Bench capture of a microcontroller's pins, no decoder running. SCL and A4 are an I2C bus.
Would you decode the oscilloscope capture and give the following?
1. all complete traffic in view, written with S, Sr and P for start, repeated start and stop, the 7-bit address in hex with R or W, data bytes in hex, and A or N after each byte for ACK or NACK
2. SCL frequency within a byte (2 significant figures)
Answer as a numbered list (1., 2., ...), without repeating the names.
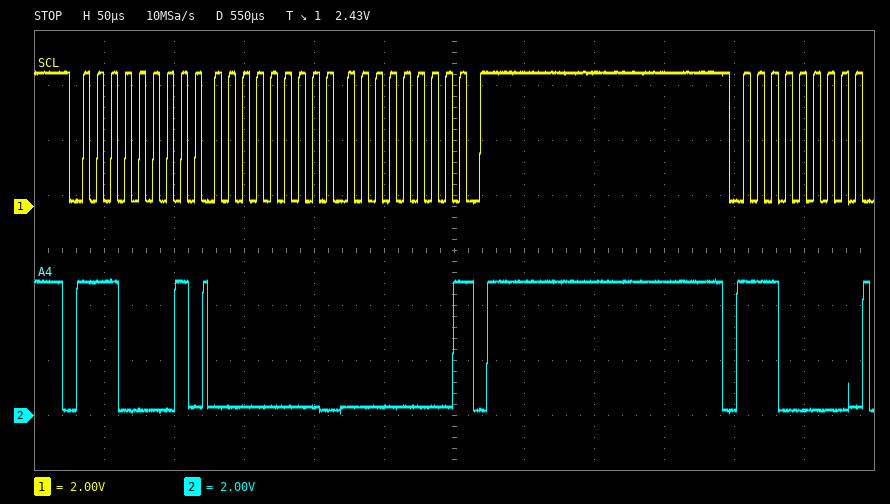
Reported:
1. S 70R A 00 A 00 N P S 70W A
2. 100 kHz
